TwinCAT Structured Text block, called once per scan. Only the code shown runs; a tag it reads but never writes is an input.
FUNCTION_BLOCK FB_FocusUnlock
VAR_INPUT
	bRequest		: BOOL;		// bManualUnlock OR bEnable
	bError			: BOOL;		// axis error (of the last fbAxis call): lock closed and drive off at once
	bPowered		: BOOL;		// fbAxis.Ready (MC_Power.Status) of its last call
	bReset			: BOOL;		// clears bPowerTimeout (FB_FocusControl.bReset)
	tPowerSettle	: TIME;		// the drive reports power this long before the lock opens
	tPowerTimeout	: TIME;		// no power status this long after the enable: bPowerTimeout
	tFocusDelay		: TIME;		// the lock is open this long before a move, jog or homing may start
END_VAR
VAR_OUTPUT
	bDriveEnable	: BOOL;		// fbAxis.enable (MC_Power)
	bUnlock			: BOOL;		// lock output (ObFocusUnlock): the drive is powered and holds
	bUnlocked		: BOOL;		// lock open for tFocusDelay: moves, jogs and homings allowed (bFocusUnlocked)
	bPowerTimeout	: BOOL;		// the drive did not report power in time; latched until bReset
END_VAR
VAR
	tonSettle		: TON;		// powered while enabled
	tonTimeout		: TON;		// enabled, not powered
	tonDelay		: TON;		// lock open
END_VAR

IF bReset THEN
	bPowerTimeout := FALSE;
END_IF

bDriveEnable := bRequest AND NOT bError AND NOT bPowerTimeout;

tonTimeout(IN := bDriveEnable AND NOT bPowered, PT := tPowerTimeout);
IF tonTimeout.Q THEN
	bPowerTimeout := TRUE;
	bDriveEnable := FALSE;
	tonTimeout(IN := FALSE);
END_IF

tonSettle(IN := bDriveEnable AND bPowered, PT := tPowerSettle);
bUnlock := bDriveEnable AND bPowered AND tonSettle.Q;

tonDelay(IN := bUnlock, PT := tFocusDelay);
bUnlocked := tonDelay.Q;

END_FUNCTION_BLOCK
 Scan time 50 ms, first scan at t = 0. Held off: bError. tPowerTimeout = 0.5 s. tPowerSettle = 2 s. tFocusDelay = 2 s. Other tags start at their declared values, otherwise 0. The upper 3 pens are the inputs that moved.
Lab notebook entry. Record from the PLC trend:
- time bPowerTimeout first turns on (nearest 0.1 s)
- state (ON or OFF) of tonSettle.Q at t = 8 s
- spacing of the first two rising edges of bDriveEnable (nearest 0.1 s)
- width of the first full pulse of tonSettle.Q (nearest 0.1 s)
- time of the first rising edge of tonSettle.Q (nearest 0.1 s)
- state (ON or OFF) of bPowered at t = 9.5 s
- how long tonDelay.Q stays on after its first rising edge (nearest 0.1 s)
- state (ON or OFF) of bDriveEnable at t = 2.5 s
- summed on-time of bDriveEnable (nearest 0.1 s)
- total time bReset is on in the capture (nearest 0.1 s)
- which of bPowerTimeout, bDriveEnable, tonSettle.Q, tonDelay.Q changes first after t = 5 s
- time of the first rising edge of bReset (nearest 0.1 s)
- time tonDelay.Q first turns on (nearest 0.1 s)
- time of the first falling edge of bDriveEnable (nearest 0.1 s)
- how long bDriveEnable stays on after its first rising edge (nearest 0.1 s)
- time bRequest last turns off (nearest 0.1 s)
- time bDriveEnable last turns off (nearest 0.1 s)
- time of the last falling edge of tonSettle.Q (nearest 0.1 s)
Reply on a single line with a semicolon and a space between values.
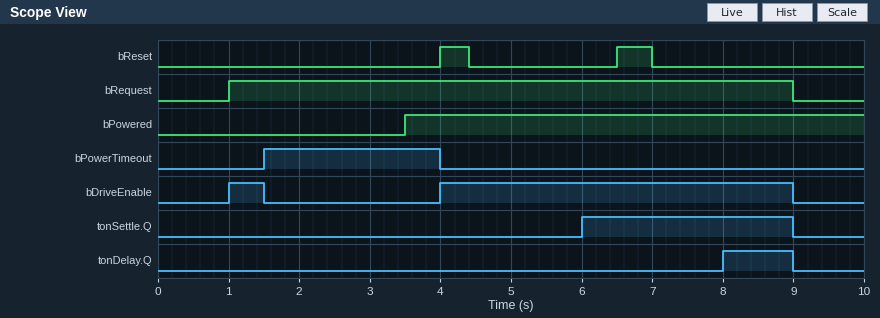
1.5 s; ON; 3.0 s; 3.0 s; 6.0 s; ON; 1.0 s; OFF; 5.5 s; 0.9 s; tonSettle.Q; 4.0 s; 8.0 s; 1.5 s; 0.5 s; 9.0 s; 9.0 s; 9.0 s
